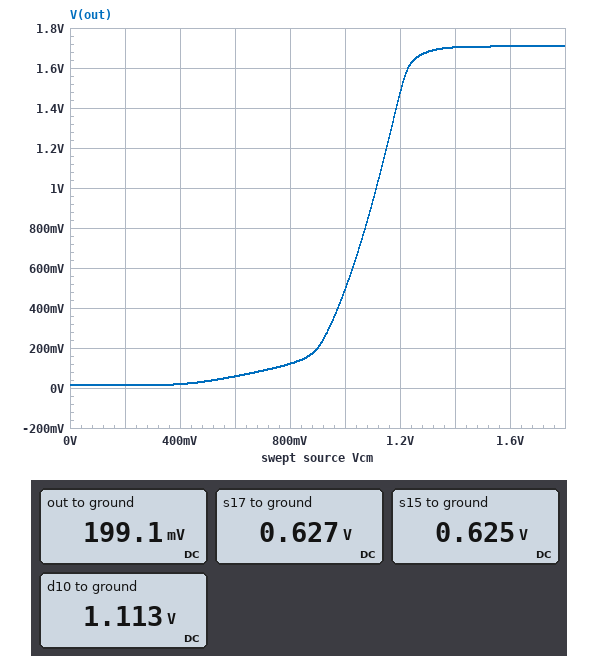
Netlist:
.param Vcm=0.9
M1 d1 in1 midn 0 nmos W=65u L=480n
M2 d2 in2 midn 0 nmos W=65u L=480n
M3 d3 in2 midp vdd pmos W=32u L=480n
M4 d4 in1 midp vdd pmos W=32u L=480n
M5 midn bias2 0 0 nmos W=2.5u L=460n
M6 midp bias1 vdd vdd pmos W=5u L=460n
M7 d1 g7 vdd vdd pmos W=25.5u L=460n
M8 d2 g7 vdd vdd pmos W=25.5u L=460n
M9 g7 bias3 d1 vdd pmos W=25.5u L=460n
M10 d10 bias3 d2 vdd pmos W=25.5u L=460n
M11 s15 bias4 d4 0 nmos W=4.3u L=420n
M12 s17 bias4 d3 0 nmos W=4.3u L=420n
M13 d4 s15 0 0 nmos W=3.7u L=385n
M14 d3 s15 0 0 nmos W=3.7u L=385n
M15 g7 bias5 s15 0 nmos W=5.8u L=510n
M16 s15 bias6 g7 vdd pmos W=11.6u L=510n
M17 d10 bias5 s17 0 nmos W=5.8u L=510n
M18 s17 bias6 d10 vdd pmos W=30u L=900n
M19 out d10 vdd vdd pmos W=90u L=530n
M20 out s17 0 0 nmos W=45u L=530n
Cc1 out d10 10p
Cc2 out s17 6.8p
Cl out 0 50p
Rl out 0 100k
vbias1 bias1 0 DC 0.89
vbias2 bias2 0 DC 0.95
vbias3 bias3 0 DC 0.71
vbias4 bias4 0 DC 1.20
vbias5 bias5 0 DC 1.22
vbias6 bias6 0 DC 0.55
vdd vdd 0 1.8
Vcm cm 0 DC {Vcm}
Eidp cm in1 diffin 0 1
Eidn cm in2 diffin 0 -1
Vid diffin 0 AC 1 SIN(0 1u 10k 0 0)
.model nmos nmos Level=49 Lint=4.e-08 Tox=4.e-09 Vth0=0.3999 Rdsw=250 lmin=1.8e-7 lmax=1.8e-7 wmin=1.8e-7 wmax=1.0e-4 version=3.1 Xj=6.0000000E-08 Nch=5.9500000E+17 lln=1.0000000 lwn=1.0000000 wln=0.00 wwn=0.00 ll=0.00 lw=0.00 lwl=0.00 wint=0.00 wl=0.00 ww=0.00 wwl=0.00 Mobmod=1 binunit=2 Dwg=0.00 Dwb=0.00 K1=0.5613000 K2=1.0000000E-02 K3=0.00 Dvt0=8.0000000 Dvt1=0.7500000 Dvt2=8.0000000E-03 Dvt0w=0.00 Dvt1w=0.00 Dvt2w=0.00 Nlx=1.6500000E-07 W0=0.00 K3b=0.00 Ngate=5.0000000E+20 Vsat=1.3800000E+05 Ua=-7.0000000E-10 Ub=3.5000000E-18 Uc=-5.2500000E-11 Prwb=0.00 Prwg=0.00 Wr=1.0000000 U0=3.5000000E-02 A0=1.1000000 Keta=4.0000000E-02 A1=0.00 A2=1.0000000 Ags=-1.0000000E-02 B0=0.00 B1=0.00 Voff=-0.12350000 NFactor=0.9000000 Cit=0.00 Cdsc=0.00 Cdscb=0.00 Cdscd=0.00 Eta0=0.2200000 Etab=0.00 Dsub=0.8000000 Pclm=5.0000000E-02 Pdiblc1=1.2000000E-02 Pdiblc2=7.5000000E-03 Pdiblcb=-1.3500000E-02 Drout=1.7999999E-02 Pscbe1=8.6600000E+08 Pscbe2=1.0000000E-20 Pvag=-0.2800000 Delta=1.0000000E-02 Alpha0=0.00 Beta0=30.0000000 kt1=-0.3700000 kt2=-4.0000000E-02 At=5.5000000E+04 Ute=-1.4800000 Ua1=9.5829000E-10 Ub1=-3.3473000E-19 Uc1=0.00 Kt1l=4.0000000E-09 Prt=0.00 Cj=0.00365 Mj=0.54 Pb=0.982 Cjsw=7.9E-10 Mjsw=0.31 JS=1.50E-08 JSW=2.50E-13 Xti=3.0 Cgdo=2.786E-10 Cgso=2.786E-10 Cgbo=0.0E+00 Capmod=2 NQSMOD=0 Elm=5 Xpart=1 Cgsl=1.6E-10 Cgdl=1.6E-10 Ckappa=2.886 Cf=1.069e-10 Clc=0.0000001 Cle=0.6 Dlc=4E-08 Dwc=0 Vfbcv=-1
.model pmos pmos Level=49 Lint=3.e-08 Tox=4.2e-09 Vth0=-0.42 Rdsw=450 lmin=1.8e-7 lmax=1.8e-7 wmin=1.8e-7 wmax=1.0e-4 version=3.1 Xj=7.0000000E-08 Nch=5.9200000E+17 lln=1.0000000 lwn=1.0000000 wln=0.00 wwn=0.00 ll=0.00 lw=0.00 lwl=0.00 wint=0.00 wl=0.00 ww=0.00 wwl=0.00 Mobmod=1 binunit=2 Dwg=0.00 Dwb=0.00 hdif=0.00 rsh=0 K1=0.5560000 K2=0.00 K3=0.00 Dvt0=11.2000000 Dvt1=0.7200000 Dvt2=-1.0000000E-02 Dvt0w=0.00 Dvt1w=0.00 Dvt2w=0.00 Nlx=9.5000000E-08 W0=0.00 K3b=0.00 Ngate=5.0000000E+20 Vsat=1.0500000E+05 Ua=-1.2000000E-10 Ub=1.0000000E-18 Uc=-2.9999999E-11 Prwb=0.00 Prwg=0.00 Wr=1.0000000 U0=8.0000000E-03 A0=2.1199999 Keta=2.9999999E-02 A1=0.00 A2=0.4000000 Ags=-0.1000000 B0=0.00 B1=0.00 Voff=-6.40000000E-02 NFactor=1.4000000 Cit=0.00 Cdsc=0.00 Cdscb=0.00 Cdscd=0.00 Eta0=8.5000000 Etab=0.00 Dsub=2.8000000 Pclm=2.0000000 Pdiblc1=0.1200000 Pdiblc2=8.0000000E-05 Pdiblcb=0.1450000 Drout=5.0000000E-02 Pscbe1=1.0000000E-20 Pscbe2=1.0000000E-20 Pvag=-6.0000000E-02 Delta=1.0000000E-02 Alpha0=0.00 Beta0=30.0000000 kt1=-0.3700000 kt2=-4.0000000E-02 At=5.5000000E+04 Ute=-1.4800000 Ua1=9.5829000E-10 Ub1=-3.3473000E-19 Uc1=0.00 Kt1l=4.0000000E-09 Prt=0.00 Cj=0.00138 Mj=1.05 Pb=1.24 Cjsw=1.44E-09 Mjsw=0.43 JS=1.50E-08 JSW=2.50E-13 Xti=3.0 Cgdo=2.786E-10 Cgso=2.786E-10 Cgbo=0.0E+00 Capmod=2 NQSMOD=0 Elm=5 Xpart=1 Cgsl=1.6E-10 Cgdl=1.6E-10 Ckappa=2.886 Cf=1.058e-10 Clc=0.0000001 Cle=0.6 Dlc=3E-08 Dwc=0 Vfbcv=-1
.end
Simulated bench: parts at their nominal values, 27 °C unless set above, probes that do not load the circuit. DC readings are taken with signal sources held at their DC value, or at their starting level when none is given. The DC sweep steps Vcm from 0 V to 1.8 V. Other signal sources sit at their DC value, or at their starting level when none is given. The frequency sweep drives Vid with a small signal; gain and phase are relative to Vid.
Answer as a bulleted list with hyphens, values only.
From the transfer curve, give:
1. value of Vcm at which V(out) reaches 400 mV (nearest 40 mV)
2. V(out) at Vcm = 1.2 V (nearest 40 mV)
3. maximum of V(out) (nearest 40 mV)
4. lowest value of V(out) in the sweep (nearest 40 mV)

- 960 mV
- 1.48 V
- 1.72 V
- 0 V
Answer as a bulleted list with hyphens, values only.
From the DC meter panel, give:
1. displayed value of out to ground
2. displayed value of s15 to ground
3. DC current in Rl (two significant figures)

- 199.1 mV
- 0.625 V
- 2.0 µA
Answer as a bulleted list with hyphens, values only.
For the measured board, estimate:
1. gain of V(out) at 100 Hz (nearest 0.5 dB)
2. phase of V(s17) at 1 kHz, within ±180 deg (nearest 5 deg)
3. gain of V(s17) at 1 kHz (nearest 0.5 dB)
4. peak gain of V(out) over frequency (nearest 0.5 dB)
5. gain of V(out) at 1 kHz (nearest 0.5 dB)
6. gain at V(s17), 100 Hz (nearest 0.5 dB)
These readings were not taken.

- 92.0 dB
- 115 deg
- 47.5 dB
- 92.0 dB
- 84.5 dB
- 55.5 dB
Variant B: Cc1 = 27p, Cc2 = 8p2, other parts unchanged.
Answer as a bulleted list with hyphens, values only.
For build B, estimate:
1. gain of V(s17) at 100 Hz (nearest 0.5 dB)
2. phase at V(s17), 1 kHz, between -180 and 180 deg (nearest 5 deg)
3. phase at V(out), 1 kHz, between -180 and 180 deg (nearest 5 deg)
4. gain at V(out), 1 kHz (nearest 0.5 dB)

- 54.5 dB
- 105 deg
- -80 deg
- 78.5 dB
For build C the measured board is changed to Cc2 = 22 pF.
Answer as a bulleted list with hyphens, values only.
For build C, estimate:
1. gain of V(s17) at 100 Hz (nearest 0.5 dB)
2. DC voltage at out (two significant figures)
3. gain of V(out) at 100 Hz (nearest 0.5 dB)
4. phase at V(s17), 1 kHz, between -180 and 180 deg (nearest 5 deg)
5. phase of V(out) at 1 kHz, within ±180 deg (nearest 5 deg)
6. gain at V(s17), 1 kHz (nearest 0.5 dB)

- 55.0 dB
- 200 mV
- 91.5 dB
- 95 deg
- -75 deg
- 43.0 dB
